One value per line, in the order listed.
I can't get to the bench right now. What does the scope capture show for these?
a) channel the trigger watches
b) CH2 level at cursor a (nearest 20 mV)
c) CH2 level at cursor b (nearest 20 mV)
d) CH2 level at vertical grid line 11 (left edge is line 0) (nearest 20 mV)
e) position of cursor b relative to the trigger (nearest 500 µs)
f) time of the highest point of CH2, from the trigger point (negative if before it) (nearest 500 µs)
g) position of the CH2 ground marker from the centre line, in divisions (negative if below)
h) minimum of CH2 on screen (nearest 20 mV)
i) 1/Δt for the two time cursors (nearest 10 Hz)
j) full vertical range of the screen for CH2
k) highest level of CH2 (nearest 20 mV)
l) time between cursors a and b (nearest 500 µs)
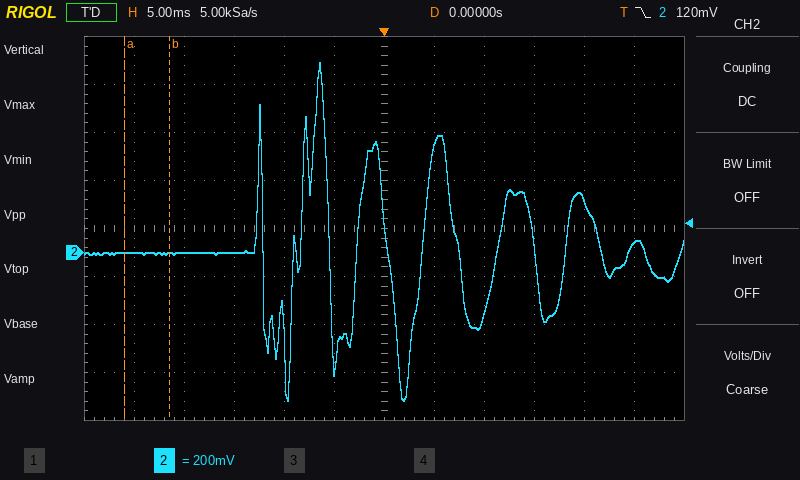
CH2
0 mV
0 mV
40 mV
-21.5 ms
-6.5 ms
-0.5 div
-620 mV
220 Hz
1.6 V
800 mV
4.5 ms
